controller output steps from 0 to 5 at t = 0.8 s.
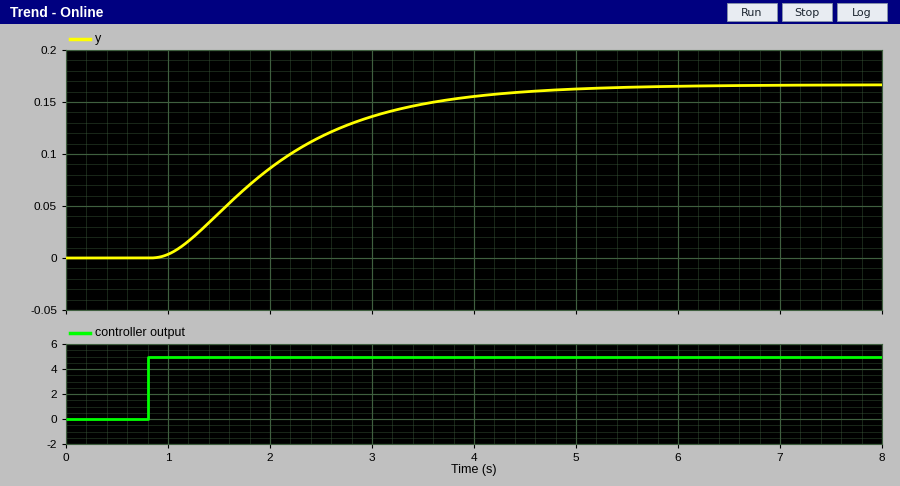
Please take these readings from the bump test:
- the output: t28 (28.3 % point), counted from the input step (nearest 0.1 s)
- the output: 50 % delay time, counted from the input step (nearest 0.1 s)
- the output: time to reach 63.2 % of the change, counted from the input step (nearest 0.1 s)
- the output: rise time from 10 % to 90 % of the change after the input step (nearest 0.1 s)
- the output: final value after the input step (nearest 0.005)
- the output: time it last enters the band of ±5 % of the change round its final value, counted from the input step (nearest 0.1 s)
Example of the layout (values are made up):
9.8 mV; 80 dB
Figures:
0.7 s; 1.2 s; 1.5 s; 2.4 s; 0.165; 3.5 s
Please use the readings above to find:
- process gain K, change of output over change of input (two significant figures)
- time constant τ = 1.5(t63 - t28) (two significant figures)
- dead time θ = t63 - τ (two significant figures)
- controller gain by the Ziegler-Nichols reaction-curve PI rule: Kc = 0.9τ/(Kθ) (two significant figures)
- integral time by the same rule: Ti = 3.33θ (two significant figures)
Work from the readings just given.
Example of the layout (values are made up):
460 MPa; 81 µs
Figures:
0.033; 1.2 s; 0.30 s; 110; 1.00 s
